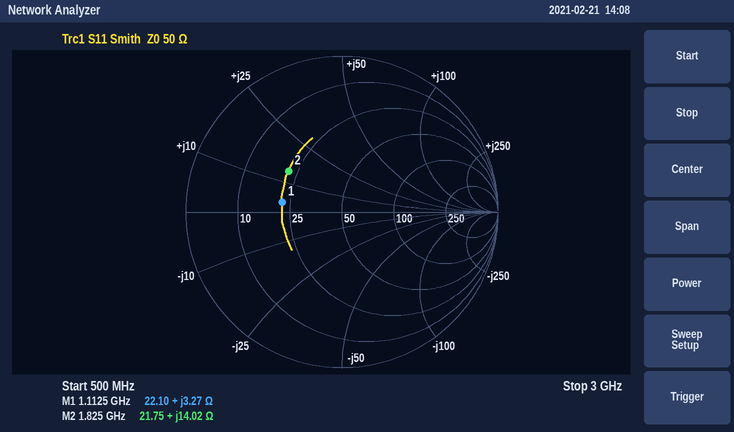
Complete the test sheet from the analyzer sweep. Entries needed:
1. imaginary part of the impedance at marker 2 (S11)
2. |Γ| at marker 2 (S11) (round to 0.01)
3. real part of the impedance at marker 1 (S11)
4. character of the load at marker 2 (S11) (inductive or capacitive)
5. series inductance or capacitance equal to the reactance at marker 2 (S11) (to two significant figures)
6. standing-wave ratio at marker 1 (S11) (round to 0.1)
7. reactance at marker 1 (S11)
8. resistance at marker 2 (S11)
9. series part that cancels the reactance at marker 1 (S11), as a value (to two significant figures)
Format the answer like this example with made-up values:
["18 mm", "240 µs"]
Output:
["+14.02 Ω", "0.43", "22.10 Ω", "inductive", "1.2 nH", "2.3", "+3.27 Ω", "21.75 Ω", "44 pF"]
